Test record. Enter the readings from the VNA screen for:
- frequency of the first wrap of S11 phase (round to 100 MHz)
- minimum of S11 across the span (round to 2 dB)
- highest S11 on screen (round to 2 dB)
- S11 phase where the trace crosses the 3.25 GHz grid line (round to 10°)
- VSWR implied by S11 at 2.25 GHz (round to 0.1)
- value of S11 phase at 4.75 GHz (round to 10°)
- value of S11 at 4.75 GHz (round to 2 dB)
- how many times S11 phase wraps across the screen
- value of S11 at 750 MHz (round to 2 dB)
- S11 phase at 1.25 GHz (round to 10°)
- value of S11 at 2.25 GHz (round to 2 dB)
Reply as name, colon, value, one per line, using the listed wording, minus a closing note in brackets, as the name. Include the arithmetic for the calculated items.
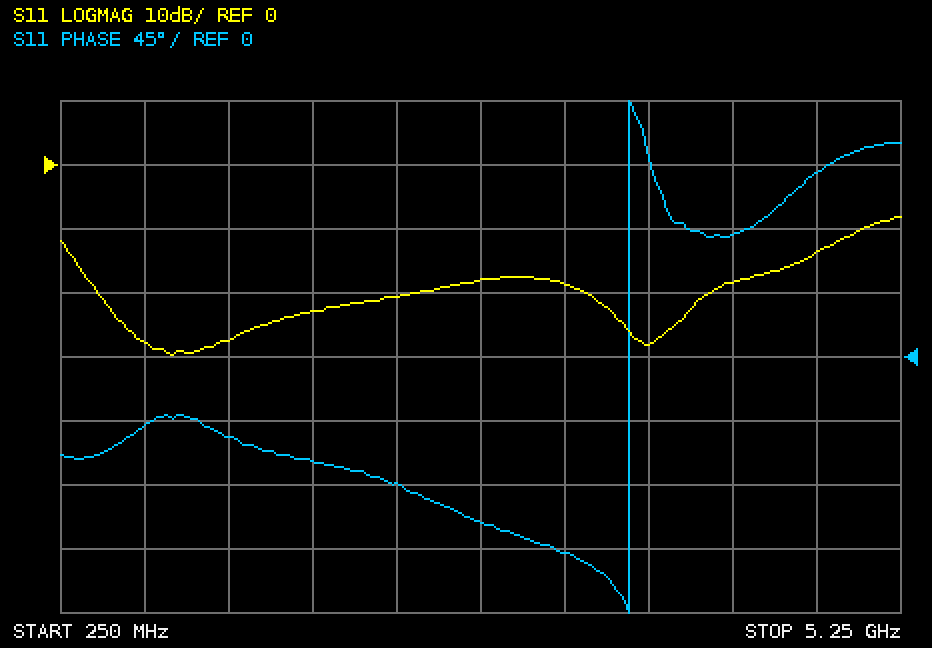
frequency of the first wrap of S11 phase: 3.6 GHz
minimum of S11 across the span: -30 dB
highest S11 on screen: -8 dB
S11 phase where the trace crosses the 3.25 GHz grid line: -140°
VSWR implied by S11 at 2.25 GHz: |Γ| = 10^(-20/20) = 0.1000; VSWR = (1 + 0.1000)/(1 − 0.1000) ≈ 1.2
value of S11 phase at 4.75 GHz: 130°
value of S11 at 4.75 GHz: -14 dB
how many times S11 phase wraps across the screen: 1
value of S11 at 750 MHz: -28 dB
S11 phase at 1.25 GHz: -60°
value of S11 at 2.25 GHz: -20 dB
